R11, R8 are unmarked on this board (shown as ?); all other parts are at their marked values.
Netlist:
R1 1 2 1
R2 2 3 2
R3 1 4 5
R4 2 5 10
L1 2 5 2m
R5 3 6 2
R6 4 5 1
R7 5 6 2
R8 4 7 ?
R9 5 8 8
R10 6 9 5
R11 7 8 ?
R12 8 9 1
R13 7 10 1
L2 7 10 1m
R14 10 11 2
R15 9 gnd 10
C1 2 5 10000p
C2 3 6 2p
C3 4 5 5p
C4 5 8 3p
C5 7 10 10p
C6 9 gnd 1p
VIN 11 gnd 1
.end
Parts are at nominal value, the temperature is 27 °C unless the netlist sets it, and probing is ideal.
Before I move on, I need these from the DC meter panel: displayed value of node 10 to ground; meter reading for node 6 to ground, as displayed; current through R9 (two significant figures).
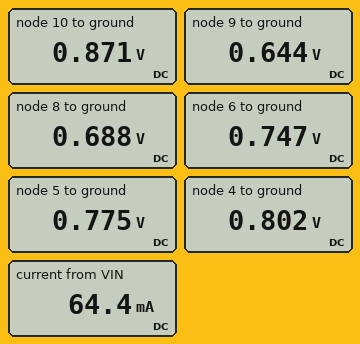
0.871 V
0.747 V
11 mA
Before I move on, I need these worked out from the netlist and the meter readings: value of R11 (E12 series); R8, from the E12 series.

5.6 Ω
2.2 Ω
